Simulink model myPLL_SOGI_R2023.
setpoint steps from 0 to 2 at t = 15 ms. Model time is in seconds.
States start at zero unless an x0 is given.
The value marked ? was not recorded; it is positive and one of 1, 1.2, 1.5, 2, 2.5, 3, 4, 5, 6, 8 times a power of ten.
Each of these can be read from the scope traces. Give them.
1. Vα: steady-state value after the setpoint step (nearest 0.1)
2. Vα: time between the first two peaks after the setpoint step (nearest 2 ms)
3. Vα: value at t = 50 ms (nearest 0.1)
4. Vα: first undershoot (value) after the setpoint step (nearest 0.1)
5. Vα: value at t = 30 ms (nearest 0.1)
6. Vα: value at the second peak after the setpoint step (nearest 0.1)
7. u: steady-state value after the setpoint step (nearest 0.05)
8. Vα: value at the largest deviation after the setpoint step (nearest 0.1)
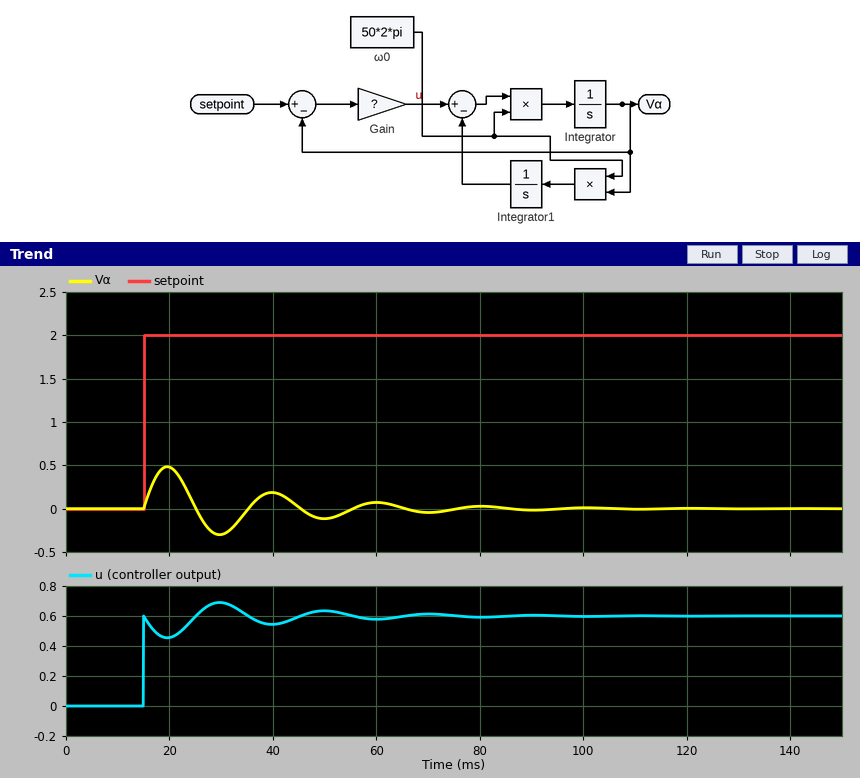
0.0
20 ms
-0.1
-0.3
-0.3
0.2
0.60
0.5
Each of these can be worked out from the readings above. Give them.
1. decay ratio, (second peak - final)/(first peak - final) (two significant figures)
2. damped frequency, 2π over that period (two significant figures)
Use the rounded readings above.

0.40
0.31 rad/ms
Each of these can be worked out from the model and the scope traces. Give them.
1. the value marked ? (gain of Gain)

0.3
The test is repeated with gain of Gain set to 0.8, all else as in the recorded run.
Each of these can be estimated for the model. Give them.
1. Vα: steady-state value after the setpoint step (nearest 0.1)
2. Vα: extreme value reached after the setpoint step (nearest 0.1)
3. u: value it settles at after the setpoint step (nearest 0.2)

0.0
1.0
1.6
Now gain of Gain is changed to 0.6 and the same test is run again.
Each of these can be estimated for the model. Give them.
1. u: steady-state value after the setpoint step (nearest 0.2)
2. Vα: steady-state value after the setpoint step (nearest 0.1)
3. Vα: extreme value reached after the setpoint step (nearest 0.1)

1.2
0.0
0.8
